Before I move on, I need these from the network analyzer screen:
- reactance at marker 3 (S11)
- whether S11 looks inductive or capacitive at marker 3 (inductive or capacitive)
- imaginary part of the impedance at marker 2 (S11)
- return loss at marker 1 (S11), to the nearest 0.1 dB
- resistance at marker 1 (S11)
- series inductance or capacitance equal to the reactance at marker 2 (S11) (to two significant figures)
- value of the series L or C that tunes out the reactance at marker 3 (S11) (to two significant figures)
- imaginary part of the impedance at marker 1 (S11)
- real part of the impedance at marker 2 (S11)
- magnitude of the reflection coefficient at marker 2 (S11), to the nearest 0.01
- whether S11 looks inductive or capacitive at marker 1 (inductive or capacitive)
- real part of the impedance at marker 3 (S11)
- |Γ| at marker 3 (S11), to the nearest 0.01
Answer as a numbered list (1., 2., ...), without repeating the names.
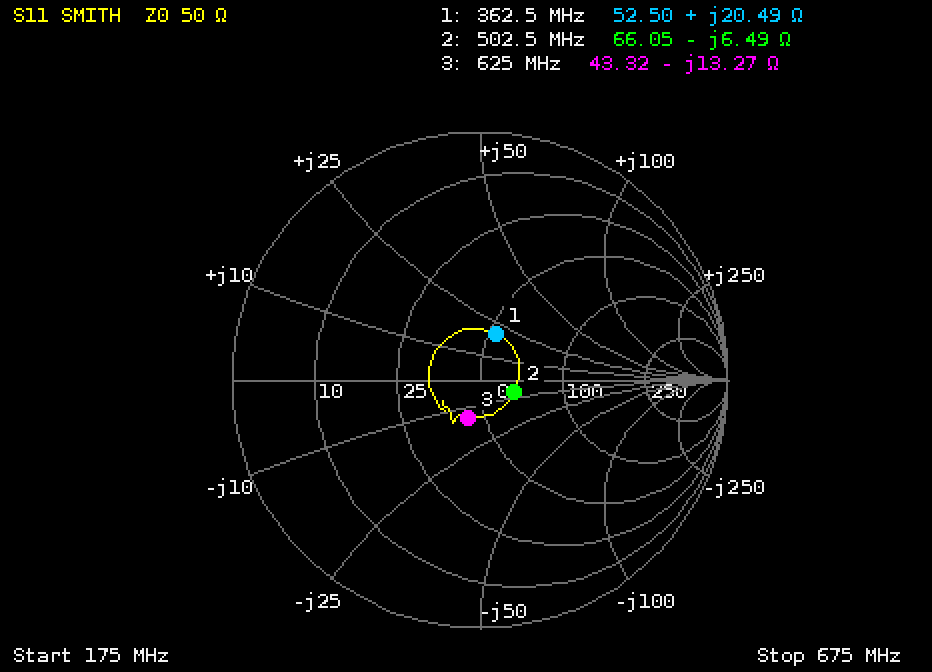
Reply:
1. -13.27 Ω
2. capacitive
3. -6.49 Ω
4. 14.1 dB
5. 52.50 Ω
6. 49 pF
7. 3.4 nH
8. +20.49 Ω
9. 66.05 Ω
10. 0.15
11. inductive
12. 43.32 Ω
13. 0.16
